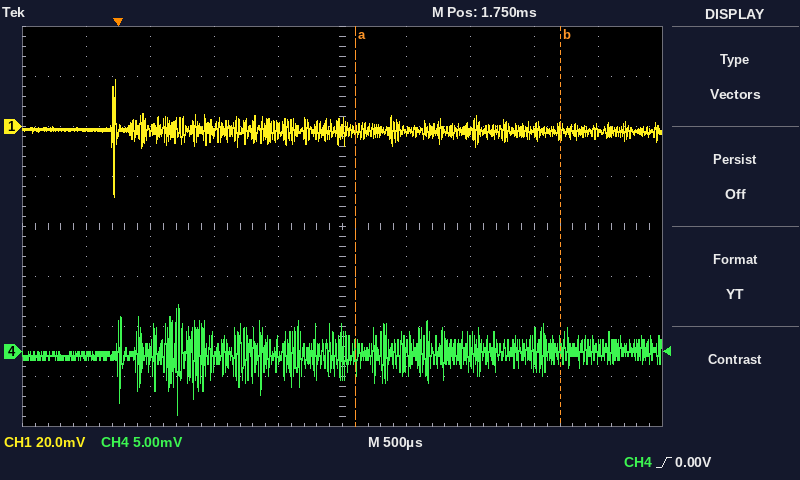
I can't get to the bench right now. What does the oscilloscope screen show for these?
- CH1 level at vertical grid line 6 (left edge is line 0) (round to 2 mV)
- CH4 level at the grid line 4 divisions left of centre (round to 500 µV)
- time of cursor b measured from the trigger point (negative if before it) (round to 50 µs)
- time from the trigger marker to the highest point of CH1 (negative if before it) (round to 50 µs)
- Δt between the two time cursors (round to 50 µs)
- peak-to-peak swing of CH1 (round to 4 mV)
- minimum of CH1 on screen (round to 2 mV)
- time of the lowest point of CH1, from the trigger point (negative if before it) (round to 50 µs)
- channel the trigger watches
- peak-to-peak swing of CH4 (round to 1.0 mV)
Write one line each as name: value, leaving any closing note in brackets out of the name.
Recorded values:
CH1 level at vertical grid line 6 (left edge is line 0): -2 mV
CH4 level at the grid line 4 divisions left of centre: -500 µV
time of cursor b measured from the trigger point (negative if before it): +3.45 ms
time from the trigger marker to the highest point of CH1 (negative if before it): 0 µs
Δt between the two time cursors: 1.60 ms
peak-to-peak swing of CH1: 48 mV
minimum of CH1 on screen: -28 mV
time of the lowest point of CH1, from the trigger point (negative if before it): -50 µs
channel the trigger watches: CH4
peak-to-peak swing of CH4: 11.0 mV
